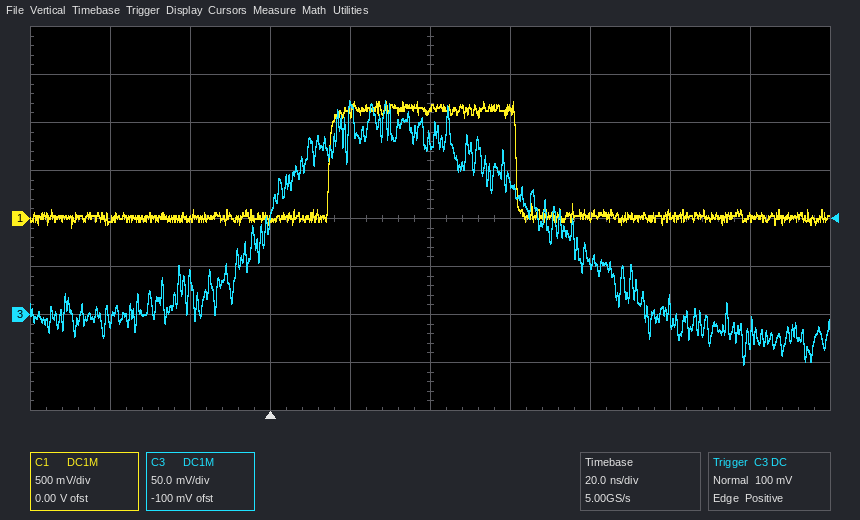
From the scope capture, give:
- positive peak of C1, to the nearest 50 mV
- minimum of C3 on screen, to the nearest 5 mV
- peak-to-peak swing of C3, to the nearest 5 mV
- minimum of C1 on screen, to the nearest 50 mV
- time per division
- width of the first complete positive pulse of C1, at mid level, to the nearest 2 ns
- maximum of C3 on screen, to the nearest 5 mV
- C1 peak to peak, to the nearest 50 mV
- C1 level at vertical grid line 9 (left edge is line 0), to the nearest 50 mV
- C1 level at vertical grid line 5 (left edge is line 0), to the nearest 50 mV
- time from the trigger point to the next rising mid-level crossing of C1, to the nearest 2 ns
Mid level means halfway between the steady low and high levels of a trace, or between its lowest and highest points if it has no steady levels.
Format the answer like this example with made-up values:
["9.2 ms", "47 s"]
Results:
["1.20 V", "-50 mV", "275 mV", "-100 mV", "20 ns", "46 ns", "225 mV", "1.30 V", "0 mV", "1.15 V", "14 ns"]
